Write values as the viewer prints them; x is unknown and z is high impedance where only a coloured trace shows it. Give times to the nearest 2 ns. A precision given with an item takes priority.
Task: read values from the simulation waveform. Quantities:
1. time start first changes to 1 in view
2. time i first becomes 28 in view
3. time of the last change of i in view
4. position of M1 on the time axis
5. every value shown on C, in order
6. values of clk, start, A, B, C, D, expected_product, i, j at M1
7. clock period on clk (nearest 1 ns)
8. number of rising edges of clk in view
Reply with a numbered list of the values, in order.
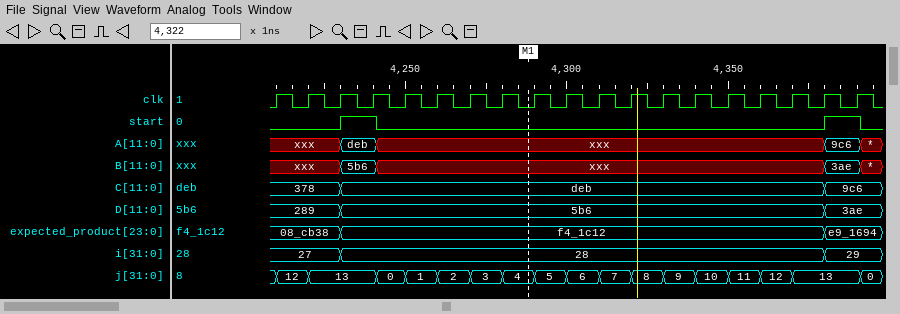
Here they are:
1. 4230 ns
2. 4230 ns
3. 4380 ns
4. 4288 ns
5. 378, deb, 9c6
6. clk=0, start=0, A=xxx, B=xxx, C=deb, D=5b6, expected_product=f4_1c12, i=28, j=4
7. 10 ns
8. 19
